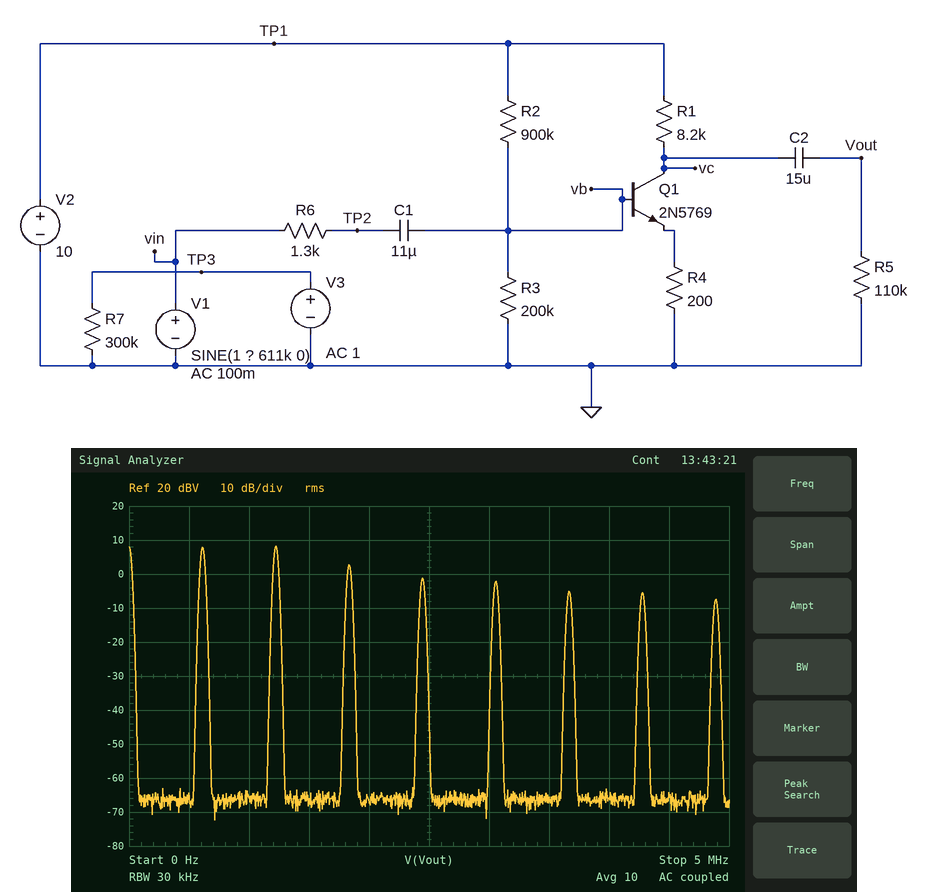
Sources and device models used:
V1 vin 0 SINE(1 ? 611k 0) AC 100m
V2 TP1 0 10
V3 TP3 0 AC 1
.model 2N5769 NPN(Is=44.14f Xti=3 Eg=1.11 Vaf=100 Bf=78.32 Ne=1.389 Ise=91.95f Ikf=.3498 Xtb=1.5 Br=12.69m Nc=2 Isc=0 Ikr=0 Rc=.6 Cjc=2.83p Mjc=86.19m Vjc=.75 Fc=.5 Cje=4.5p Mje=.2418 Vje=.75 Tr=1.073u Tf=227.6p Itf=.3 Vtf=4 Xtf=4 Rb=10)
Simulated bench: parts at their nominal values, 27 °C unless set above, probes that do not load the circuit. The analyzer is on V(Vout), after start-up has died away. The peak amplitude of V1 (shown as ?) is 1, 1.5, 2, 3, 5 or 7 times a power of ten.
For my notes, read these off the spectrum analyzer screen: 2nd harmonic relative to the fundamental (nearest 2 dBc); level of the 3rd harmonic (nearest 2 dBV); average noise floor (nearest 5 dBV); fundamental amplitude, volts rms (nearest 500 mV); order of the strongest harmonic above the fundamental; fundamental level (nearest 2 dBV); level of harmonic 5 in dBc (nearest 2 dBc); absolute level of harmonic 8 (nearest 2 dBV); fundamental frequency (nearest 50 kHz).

0 dBc
2 dBV
-65 dBV
2.5 V
2
8 dBV
-10 dBc
-8 dBV
600 kHz
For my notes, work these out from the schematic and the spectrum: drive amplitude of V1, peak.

100 V
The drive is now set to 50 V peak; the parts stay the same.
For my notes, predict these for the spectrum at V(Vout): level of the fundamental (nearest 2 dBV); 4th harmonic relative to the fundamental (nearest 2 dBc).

8 dBV
-14 dBc
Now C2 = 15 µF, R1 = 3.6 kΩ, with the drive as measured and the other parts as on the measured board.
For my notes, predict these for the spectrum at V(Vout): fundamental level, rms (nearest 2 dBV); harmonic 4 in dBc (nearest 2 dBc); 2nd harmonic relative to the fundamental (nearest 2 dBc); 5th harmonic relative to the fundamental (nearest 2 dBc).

2 dBV
-8 dBc
4 dBc
-4 dBc
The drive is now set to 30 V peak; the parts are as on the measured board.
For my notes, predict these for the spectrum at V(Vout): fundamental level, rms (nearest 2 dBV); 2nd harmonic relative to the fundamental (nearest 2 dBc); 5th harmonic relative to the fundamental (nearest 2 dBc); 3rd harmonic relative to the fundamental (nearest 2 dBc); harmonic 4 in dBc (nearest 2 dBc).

10 dBV
-12 dBc
-12 dBc
-6 dBc
-20 dBc
